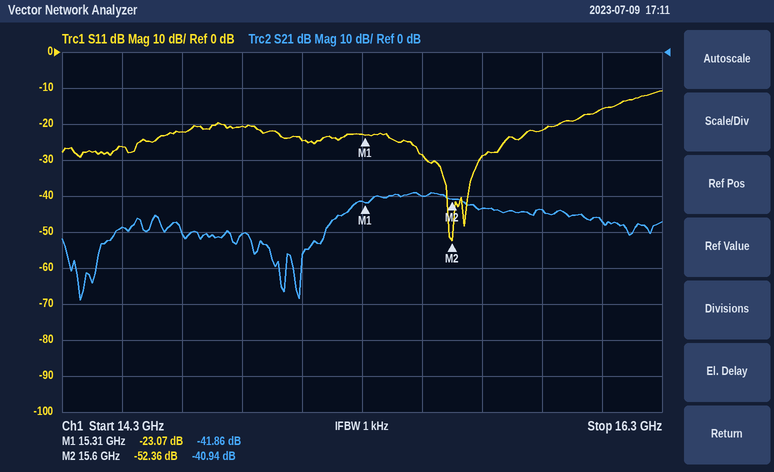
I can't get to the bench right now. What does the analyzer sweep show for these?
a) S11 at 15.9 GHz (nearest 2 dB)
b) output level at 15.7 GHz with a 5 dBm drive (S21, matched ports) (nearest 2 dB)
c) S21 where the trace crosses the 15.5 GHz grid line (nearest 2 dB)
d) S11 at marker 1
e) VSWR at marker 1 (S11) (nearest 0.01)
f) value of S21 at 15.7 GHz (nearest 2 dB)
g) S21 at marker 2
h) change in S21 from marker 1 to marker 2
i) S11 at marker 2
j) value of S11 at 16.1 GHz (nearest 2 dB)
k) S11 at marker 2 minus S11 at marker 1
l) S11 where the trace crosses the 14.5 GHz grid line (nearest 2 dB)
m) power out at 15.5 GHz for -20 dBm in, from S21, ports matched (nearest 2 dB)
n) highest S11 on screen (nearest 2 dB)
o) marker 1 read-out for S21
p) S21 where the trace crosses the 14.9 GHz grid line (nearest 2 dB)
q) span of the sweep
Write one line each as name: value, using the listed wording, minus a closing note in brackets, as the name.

S11 at 15.9 GHz: -22 dB
output level at 15.7 GHz with a 5 dBm drive (S21, matched ports): -38 dBm
S21 where the trace crosses the 15.5 GHz grid line: -40 dB
S11 at marker 1: -23.07 dB
VSWR at marker 1 (S11): 1.15
value of S21 at 15.7 GHz: -44 dB
S21 at marker 2: -40.94 dB
change in S21 from marker 1 to marker 2: 0.92 dB
S11 at marker 2: -52.36 dB
value of S11 at 16.1 GHz: -16 dB
S11 at marker 2 minus S11 at marker 1: -29.29 dB
S11 where the trace crosses the 14.5 GHz grid line: -26 dB
power out at 15.5 GHz for -20 dBm in, from S21, ports matched: -60 dBm
highest S11 on screen: -10 dB
marker 1 read-out for S21: -41.86 dB
S21 where the trace crosses the 14.9 GHz grid line: -50 dB
span of the sweep: 2 GHz
